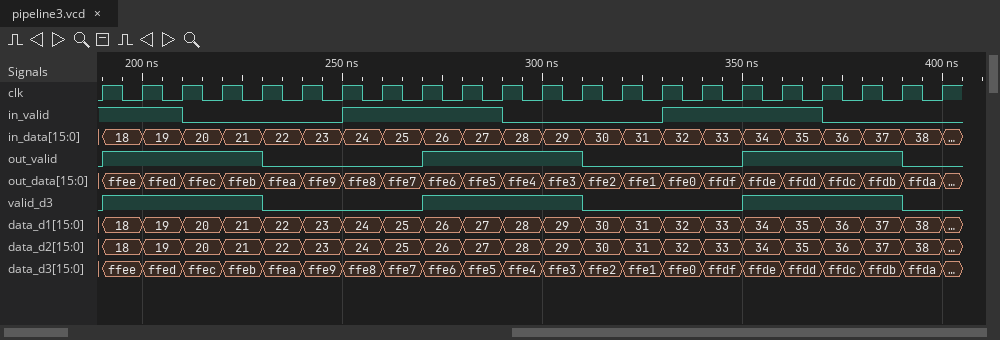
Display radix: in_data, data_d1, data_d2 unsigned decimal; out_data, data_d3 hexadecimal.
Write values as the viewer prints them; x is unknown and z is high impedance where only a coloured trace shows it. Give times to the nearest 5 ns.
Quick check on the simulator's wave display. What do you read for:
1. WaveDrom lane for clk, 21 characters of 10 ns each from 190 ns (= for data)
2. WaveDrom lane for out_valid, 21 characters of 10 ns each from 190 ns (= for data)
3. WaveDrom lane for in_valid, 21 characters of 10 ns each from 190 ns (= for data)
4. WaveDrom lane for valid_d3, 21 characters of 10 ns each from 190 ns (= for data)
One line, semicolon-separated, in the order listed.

{name: 'clk', wave: 'p....................'}; {name: 'out_valid', wave: '1...0...1...0...1...0'}; {name: 'in_valid', wave: '1.0...1...0...1...0..'}; {name: 'valid_d3', wave: '1...0...1...0...1...0'}
